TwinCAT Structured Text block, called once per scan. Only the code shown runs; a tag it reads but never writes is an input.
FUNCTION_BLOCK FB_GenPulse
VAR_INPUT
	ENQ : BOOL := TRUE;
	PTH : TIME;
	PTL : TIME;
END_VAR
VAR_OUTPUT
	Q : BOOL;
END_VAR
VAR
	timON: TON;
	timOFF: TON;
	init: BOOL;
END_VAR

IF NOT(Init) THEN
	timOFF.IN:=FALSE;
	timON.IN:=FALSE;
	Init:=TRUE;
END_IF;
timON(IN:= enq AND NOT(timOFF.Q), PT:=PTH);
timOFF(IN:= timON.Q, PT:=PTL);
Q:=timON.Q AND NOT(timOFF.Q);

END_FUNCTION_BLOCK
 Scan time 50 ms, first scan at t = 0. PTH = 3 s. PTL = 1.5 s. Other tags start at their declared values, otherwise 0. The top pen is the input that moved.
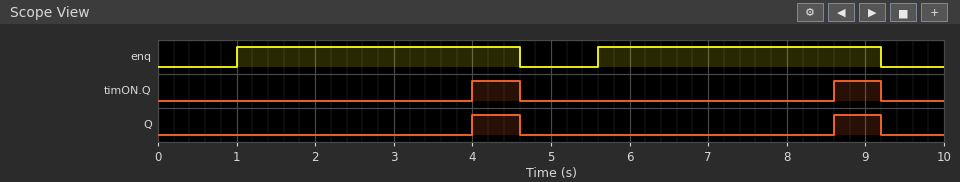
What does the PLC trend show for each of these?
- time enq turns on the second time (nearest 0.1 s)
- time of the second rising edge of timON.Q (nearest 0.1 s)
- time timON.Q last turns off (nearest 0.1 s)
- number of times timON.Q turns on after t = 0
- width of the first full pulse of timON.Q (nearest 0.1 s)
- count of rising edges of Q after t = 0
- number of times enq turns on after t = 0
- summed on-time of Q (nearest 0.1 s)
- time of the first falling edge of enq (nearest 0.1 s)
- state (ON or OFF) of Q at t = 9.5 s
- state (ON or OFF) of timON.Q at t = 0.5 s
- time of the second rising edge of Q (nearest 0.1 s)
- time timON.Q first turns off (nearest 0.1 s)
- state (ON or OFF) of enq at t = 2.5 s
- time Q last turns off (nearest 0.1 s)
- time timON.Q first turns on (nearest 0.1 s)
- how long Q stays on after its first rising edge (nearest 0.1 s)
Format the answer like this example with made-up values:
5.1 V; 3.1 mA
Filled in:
5.6 s; 8.6 s; 9.2 s; 2; 0.6 s; 2; 2; 1.2 s; 4.6 s; OFF; OFF; 8.6 s; 4.6 s; ON; 9.2 s; 4.0 s; 0.6 s
